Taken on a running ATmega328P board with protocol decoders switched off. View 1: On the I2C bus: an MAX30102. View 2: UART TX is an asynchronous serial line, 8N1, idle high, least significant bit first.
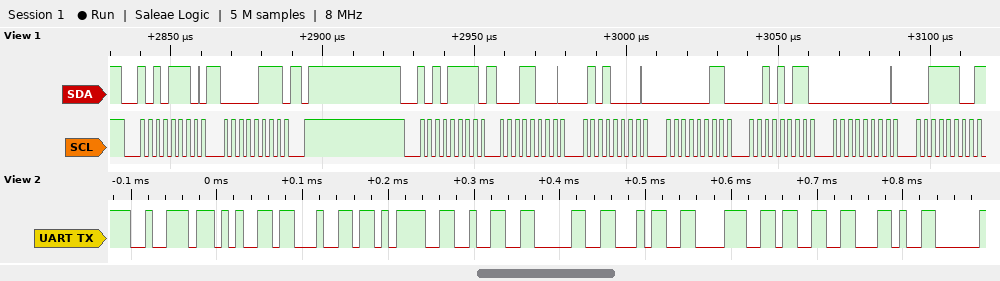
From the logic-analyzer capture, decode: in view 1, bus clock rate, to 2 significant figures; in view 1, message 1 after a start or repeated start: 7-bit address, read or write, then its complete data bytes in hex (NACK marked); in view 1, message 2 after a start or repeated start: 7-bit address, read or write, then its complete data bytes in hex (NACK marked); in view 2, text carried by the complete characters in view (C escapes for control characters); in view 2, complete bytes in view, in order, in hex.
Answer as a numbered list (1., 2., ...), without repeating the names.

1. 400 kHz
2. 0x57 write: 07
3. 0x57 read: 18 50 03 2B 00 3C NACK
4. "red=20483,"
5. 72 65 64 3D 32 30 34 38 33 2C
